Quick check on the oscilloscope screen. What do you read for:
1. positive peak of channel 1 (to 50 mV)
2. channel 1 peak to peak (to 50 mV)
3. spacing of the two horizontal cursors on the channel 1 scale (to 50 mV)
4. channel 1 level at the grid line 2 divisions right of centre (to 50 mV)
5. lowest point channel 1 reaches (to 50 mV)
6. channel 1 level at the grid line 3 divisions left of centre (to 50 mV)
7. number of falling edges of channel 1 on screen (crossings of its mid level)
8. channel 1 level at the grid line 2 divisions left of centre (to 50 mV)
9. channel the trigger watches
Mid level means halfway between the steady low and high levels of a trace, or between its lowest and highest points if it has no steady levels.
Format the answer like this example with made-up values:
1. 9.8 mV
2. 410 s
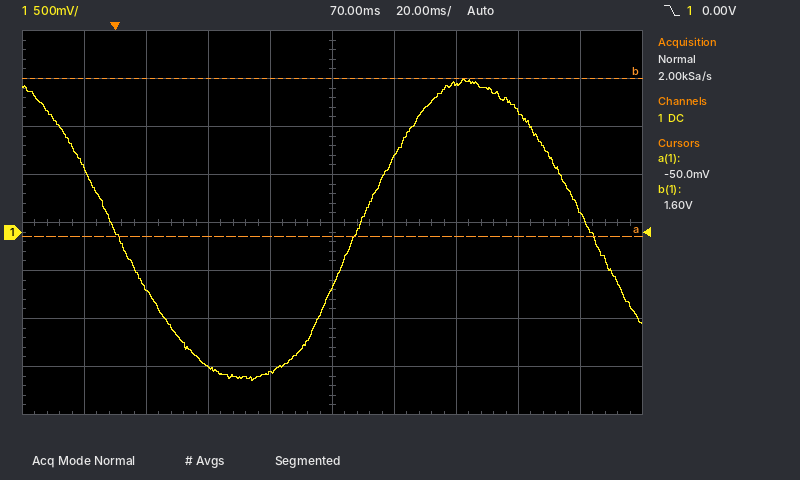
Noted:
1. 1.60 V
2. 3.15 V
3. 1.65 V
4. 1.55 V
5. -1.55 V
6. -600 mV
7. 2
8. -1.40 V
9. channel 1
